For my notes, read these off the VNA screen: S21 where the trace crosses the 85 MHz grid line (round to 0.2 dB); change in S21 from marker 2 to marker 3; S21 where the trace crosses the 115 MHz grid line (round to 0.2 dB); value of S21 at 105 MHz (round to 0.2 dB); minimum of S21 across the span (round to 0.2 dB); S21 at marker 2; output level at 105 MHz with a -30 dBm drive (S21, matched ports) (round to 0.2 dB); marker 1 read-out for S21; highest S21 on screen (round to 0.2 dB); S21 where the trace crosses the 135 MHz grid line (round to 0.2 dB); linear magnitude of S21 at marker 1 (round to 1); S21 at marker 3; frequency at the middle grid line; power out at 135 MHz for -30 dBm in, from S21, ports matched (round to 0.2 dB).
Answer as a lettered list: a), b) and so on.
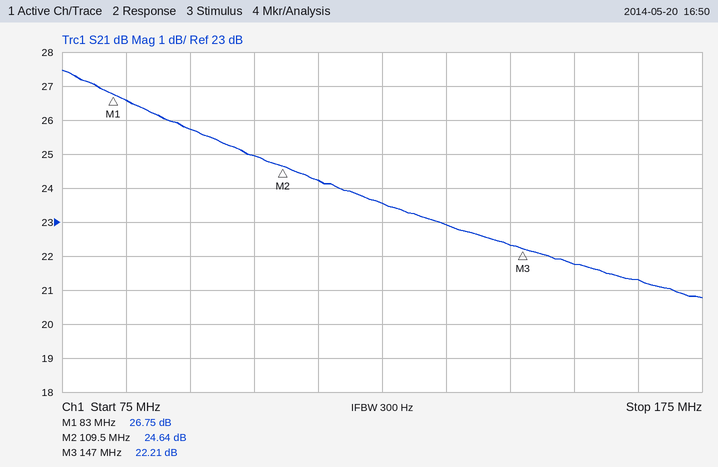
a) 26.6 dB
b) -2.43 dB
c) 24.2 dB
d) 25.0 dB
e) 20.8 dB
f) 24.64 dB
g) -5.0 dBm
h) 26.75 dB
i) 27.4 dB
j) 23.0 dB
k) 22
l) 22.21 dB
m) 125 MHz
n) -7.0 dBm
